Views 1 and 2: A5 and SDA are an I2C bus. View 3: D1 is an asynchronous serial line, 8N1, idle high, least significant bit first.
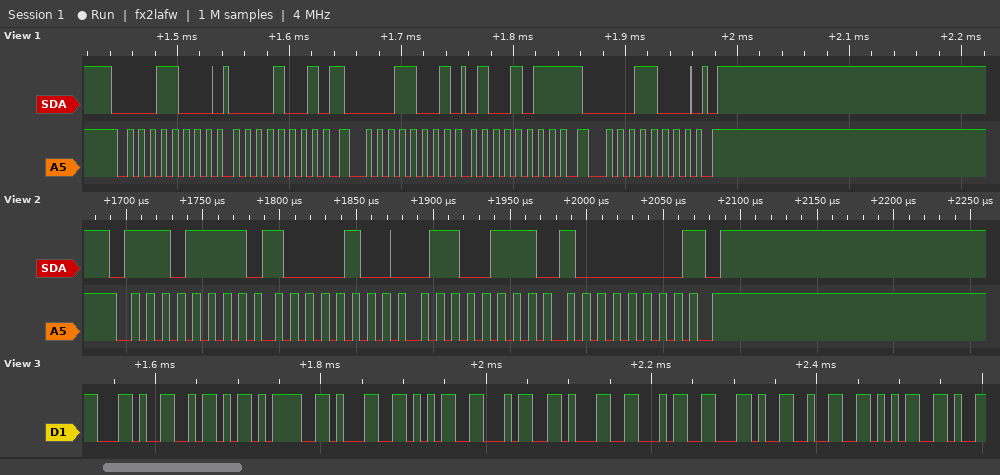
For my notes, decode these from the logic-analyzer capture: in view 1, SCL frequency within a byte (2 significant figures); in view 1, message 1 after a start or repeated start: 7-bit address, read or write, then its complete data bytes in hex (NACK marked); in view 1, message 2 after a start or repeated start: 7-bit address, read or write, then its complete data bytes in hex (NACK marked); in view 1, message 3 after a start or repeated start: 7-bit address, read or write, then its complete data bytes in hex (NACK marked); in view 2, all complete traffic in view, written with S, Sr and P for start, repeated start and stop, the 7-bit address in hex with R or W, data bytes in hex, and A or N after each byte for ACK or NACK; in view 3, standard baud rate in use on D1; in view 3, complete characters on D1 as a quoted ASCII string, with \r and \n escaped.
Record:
100 kHz
0x0C write: 09
0x0C read: 4B NACK
0x0C write
S 77R A 84 A 67 A 80 N P
115200 baud
",Z=15414,25"
